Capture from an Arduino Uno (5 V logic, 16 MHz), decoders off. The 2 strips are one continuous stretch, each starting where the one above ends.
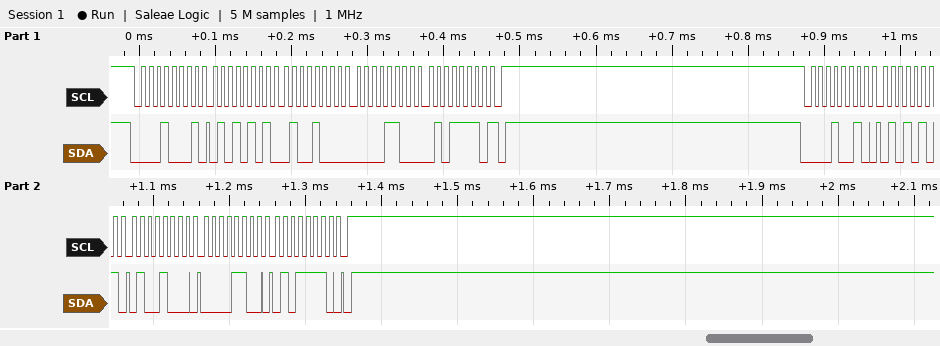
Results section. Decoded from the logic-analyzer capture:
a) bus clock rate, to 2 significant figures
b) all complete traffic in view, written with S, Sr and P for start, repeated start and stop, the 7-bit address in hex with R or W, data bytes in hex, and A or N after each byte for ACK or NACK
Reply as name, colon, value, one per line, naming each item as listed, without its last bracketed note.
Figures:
bus clock rate, to 2 significant figures: 100 kHz
all complete traffic in view, written with S, Sr and P for start, repeated start and stop, the 7-bit address in hex with R or W, data bytes in hex, and A or N after each byte for ACK or NACK: S 08R A 55 A 48 A 0C A 5E N P S 09W A 55 A 48 A 0C A 5E A P
